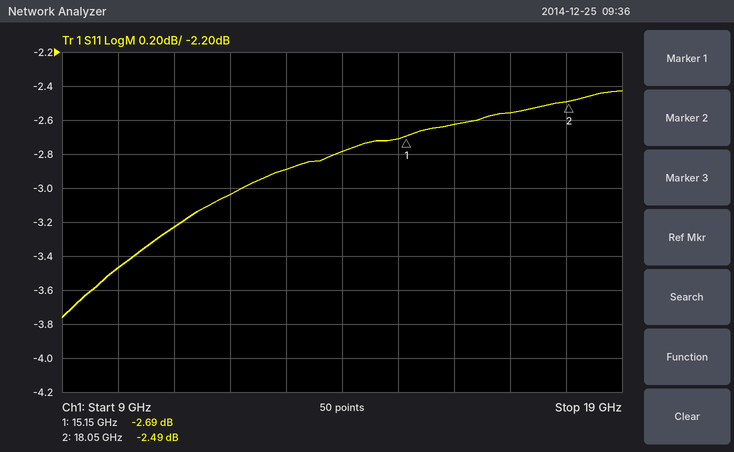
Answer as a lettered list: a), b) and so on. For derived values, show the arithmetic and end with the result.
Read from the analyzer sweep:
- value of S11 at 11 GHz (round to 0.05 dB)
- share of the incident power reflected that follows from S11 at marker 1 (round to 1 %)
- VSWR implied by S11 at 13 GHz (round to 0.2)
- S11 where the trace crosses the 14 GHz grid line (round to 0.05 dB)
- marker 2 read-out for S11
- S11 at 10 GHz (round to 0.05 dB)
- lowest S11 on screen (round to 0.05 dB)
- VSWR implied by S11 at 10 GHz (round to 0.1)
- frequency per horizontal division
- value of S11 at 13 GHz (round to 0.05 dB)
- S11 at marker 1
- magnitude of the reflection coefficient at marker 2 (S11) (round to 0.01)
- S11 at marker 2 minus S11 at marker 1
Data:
a) -3.25 dB
b) 10^(-2.69/10) ≈ 54 %
c) |Γ| = 10^(-2.9/20) = 0.7161; VSWR = (1 + 0.7161)/(1 − 0.7161) ≈ 6.0
d) -2.80 dB
e) -2.49 dB
f) -3.45 dB
g) -3.75 dB
h) |Γ| = 10^(-3.45/20) = 0.6722; VSWR = (1 + 0.6722)/(1 − 0.6722) ≈ 5.1
i) 1 GHz
j) -2.90 dB
k) -2.69 dB
l) 10^(-2.49/20) ≈ 0.75
m) -2.49 − (-2.69) = 0.20 dB
